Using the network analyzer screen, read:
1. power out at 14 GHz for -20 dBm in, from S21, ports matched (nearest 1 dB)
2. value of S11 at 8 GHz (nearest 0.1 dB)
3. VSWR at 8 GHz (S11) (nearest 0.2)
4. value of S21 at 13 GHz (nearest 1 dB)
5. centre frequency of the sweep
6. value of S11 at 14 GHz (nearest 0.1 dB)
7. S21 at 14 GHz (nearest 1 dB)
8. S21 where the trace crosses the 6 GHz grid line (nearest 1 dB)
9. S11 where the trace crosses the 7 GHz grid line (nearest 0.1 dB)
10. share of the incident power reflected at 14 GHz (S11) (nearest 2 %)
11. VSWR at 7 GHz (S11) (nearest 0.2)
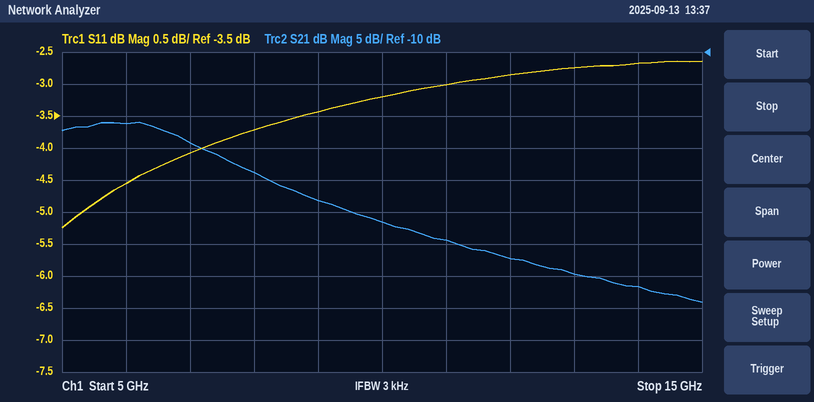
-67 dBm
-3.7 dB
4.8
-45 dB
10 GHz
-2.7 dB
-47 dB
-21 dB
-4.1 dB
54 %
4.4
